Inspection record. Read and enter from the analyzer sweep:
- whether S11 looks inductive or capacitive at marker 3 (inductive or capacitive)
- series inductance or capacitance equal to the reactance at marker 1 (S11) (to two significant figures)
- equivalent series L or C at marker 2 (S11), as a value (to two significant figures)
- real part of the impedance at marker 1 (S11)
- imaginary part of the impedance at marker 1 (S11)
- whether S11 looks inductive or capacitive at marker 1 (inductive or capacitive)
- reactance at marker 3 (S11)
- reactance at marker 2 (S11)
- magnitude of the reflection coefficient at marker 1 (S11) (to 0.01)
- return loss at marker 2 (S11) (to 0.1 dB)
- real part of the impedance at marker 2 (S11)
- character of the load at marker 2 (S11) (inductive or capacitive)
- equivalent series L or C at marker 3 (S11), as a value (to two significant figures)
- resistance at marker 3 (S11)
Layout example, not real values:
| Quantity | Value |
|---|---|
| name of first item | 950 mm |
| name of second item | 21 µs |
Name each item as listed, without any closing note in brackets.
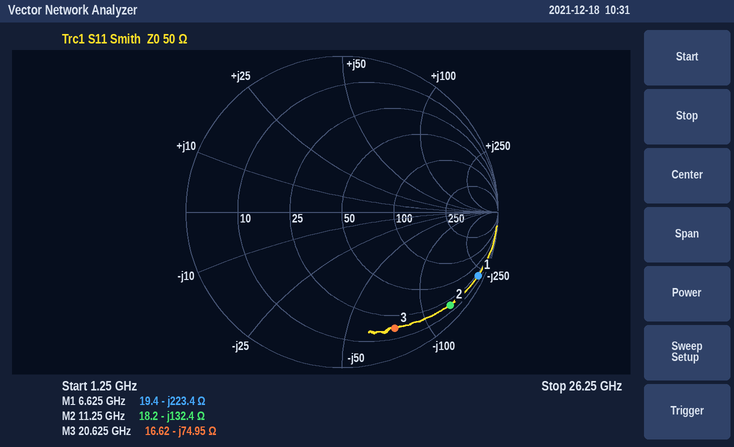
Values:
| Quantity | Value |
|---|---|
| whether S11 looks inductive or capacitive at marker 3 | capacitive |
| series inductance or capacitance equal to the reactance at marker 1 (S11) | 110 fF |
| equivalent series L or C at marker 2 (S11), as a value | 110 fF |
| real part of the impedance at marker 1 | 19.4 Ω |
| imaginary part of the impedance at marker 1 | -223.4 Ω |
| whether S11 looks inductive or capacitive at marker 1 | capacitive |
| reactance at marker 3 | -74.95 Ω |
| reactance at marker 2 | -132.4 Ω |
| magnitude of the reflection coefficient at marker 1 (S11) | 0.96 |
| return loss at marker 2 (S11) | 0.8 dB |
| real part of the impedance at marker 2 | 18.2 Ω |
| character of the load at marker 2 (S11) | capacitive |
| equivalent series L or C at marker 3 (S11), as a value | 100 fF |
| resistance at marker 3 | 16.62 Ω |
